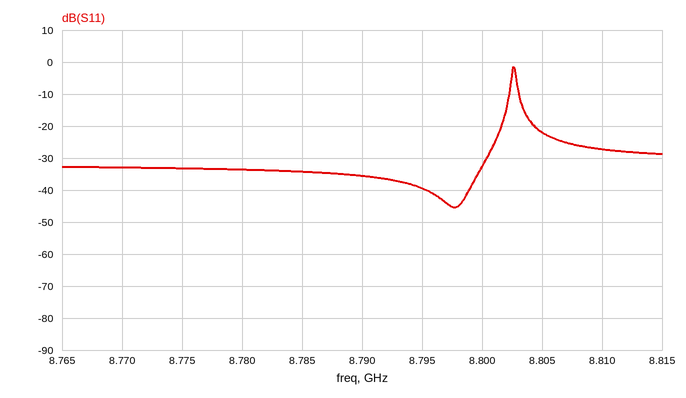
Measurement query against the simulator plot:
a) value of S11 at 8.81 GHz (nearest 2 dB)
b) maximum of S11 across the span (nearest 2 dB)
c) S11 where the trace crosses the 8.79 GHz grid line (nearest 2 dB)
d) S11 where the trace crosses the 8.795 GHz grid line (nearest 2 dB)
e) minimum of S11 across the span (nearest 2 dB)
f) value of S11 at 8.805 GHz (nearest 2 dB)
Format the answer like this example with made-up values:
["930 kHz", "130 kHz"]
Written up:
["-28 dB", "-2 dB", "-36 dB", "-40 dB", "-46 dB", "-22 dB"]
